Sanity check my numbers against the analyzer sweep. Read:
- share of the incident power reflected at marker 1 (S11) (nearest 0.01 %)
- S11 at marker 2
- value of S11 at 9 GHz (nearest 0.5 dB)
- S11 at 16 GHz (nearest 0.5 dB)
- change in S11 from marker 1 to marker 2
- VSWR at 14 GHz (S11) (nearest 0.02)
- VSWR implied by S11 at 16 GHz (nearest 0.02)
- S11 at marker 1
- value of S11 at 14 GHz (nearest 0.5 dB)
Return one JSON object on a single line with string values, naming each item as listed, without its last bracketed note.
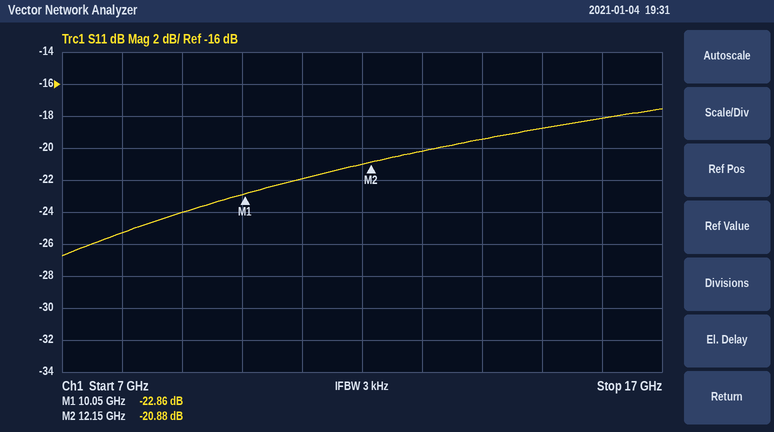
{"share of the incident power reflected at marker 1 (S11)": "0.52 %", "S11 at marker 2": "-20.88 dB", "value of S11 at 9 GHz": "-24.0 dB", "S11 at 16 GHz": "-18.0 dB", "change in S11 from marker 1 to marker 2": "1.98 dB", "VSWR at 14 GHz (S11)": "1.24", "VSWR implied by S11 at 16 GHz": "1.28", "S11 at marker 1": "-22.86 dB", "value of S11 at 14 GHz": "-19.5 dB"}
